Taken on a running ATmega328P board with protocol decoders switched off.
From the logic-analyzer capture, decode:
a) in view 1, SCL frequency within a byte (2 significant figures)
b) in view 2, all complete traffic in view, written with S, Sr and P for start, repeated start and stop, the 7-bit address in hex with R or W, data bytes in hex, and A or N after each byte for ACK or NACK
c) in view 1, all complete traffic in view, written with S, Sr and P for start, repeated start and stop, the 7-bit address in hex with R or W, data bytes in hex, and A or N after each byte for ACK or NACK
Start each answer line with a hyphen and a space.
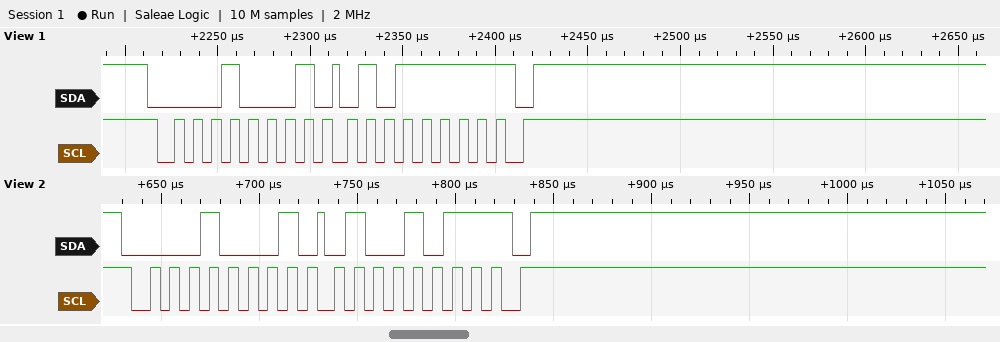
- 100 kHz
- S 08R A 4B N P
- S 08R A 5F N P
